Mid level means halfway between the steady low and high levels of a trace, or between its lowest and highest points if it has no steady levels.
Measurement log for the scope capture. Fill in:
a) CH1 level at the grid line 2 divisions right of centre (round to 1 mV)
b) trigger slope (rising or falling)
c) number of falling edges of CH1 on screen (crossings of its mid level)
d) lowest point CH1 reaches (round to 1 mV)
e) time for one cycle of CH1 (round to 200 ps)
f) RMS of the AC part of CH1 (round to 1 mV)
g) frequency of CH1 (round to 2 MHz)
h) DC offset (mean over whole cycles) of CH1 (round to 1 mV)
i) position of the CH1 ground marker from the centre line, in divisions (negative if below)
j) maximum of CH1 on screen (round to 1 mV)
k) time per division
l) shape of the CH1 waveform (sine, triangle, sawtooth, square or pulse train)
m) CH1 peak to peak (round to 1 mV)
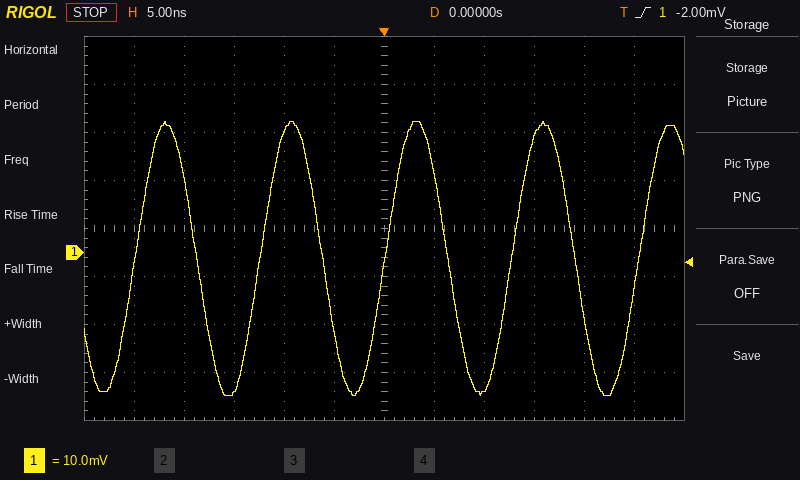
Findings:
-29 mV
rising
4
-30 mV
12.6 ns
20 mV
80 MHz
-1 mV
-0.5 div
27 mV
5 ns
sine
57 mV
